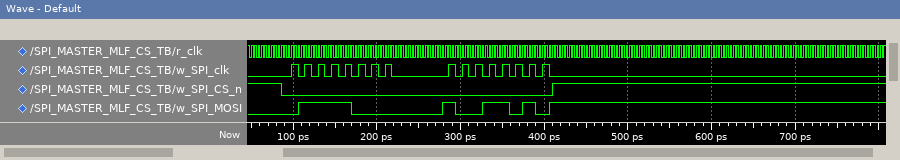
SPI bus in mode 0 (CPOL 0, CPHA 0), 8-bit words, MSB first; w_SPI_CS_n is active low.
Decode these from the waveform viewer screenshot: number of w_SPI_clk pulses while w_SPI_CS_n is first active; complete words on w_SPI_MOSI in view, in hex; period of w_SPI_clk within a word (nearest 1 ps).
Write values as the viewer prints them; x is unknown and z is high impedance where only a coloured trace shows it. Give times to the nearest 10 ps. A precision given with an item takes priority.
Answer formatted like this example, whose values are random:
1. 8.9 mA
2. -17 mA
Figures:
1. 16
2. 78, 9A
3. 16 ps
